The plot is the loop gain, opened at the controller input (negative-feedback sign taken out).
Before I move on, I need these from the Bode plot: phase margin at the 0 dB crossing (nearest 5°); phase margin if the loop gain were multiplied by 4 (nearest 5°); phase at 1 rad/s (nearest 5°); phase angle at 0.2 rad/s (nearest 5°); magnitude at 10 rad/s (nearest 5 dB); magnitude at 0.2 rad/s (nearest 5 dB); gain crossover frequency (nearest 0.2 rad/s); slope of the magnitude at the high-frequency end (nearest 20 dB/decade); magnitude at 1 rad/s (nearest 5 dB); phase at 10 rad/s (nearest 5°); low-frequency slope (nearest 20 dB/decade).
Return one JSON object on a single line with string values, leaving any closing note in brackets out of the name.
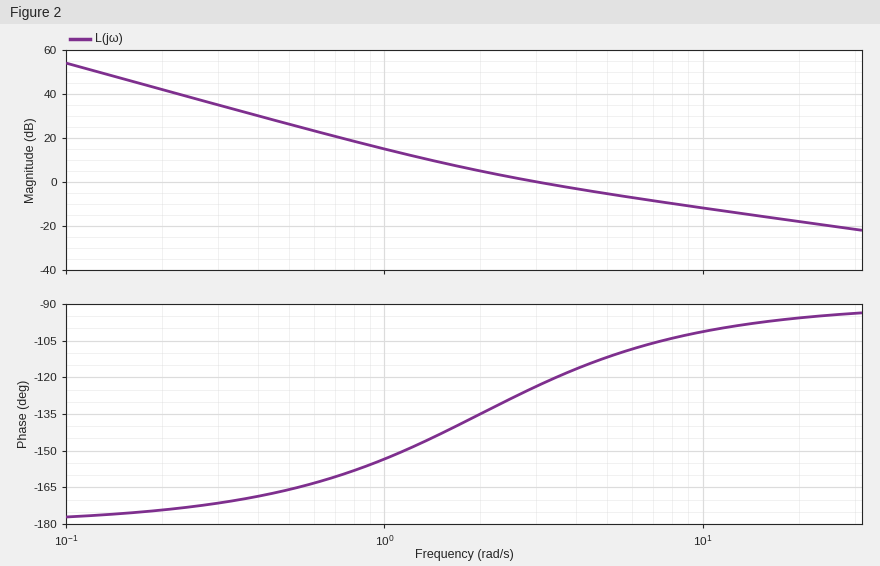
{"phase margin at the 0 dB crossing": "55°", "phase margin if the loop gain were multiplied by 4": "80°", "phase at 1 rad/s": "-155°", "phase angle at 0.2 rad/s": "-175°", "magnitude at 10 rad/s": "-10 dB", "magnitude at 0.2 rad/s": "40 dB", "gain crossover frequency": "3.0 rad/s", "slope of the magnitude at the high-frequency end": "-20 dB/decade", "magnitude at 1 rad/s": "15 dB", "phase at 10 rad/s": "-100°", "low-frequency slope": "-40 dB/decade"}
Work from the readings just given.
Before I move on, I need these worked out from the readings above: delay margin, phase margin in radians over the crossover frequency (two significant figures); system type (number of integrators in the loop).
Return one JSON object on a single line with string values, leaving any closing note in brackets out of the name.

{"delay margin, phase margin in radians over the crossover frequency": "0.32 s", "system type": "2"}
